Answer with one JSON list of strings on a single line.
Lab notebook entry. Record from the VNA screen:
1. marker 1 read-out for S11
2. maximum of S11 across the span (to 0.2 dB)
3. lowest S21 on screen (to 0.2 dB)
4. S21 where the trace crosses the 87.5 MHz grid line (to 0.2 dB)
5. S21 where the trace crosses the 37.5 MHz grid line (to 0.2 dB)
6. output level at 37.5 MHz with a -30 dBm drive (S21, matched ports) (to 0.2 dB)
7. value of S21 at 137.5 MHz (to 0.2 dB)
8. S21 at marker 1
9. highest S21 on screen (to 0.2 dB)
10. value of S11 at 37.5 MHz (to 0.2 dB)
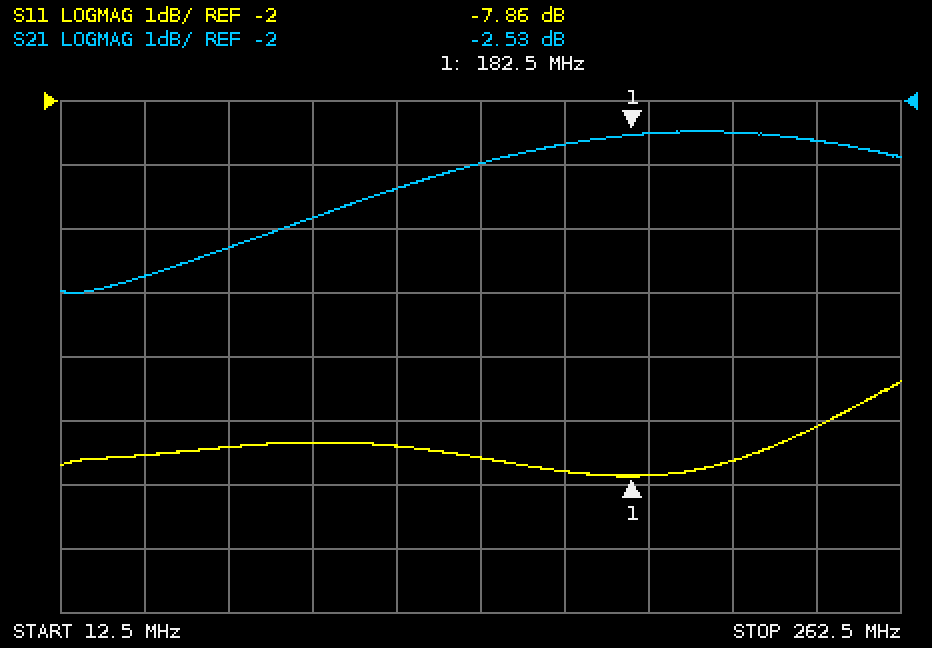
["-7.86 dB", "-6.4 dB", "-5.0 dB", "-3.8 dB", "-4.8 dB", "-34.8 dBm", "-3.0 dB", "-2.53 dB", "-2.4 dB", "-7.6 dB"]
